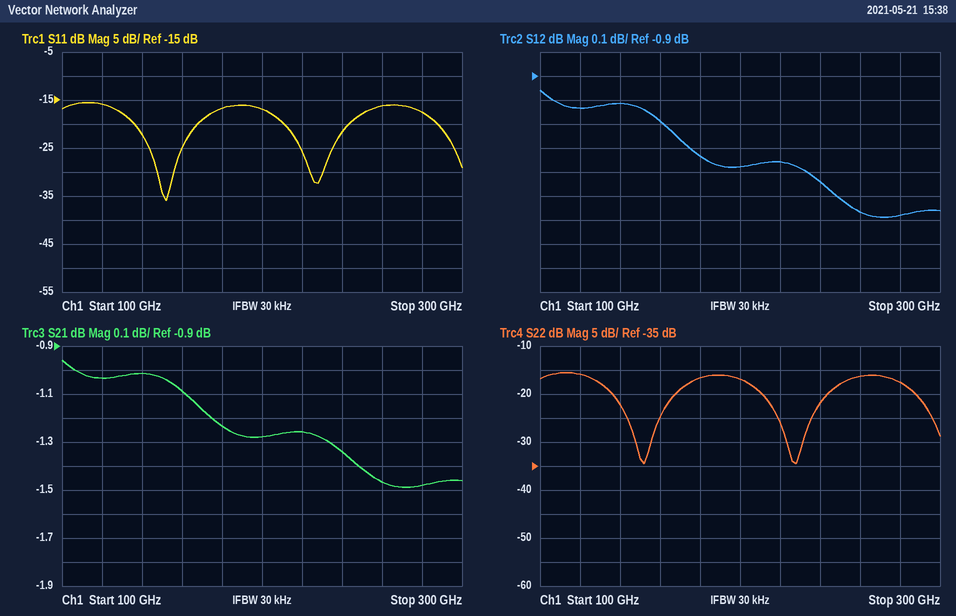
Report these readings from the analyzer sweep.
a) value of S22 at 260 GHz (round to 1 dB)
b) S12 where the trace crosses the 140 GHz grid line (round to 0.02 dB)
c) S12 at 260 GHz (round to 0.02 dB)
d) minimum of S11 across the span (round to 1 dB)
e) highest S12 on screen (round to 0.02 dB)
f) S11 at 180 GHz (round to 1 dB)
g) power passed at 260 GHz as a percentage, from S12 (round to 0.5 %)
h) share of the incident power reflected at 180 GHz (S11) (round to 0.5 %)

-16 dB
-1.02 dB
-1.46 dB
-36 dB
-0.96 dB
-17 dB
71.5 %
2.0 %
